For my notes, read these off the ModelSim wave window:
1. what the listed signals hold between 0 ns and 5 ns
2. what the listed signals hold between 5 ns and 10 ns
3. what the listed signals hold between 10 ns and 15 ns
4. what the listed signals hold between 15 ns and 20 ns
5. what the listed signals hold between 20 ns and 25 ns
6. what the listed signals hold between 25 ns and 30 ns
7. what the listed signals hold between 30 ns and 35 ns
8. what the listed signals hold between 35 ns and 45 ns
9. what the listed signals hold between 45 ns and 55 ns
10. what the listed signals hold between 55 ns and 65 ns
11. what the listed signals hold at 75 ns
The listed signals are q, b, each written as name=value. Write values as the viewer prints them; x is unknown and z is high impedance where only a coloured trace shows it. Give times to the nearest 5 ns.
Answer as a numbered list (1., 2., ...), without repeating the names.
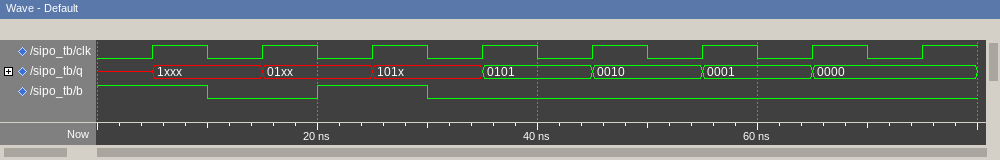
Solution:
1. q=x, b=1
2. q=1xxx, b=1
3. q=1xxx, b=0
4. q=01xx, b=0
5. q=01xx, b=1
6. q=101x, b=1
7. q=101x, b=0
8. q=0101, b=0
9. q=0010, b=0
10. q=0001, b=0
11. q=0000, b=0
